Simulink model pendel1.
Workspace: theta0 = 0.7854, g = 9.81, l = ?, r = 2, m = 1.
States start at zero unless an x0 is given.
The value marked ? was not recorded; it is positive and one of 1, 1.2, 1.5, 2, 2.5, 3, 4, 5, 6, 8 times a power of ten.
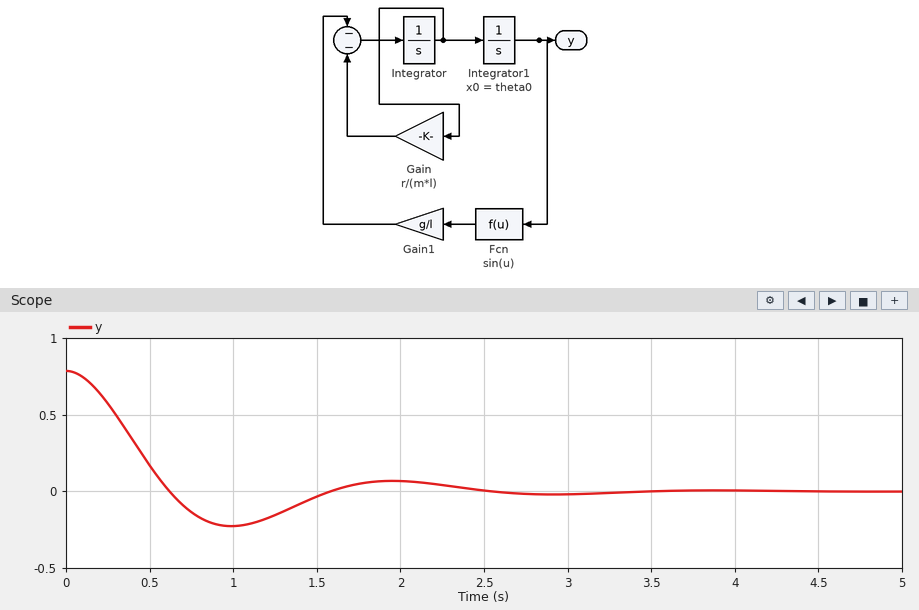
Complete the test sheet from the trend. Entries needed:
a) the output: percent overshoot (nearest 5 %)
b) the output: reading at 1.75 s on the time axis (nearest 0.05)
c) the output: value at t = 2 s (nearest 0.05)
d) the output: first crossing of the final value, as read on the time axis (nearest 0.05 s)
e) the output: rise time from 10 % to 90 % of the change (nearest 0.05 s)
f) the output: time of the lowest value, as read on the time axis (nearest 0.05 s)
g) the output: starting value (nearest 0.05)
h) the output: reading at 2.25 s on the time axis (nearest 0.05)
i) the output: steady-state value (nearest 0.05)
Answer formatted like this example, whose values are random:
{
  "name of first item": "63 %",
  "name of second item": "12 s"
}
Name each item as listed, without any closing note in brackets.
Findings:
{
  "the output: percent overshoot": "30 %",
  "the output: reading at 1.75 s on the time axis": "0.05",
  "the output: value at t = 2 s": "0.05",
  "the output: first crossing of the final value, as read on the time axis": "0.60 s",
  "the output: rise time from 10 % to 90 % of the change": "0.40 s",
  "the output: time of the lowest value, as read on the time axis": "1.00 s",
  "the output: starting value": "0.80",
  "the output: reading at 2.25 s on the time axis": "0.05",
  "the output: steady-state value": "0.00"
}
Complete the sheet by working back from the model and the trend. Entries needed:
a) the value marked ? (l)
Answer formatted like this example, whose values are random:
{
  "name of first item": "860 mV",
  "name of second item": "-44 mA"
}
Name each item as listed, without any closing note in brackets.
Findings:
{
  "the value marked ?": "0.8"
}
